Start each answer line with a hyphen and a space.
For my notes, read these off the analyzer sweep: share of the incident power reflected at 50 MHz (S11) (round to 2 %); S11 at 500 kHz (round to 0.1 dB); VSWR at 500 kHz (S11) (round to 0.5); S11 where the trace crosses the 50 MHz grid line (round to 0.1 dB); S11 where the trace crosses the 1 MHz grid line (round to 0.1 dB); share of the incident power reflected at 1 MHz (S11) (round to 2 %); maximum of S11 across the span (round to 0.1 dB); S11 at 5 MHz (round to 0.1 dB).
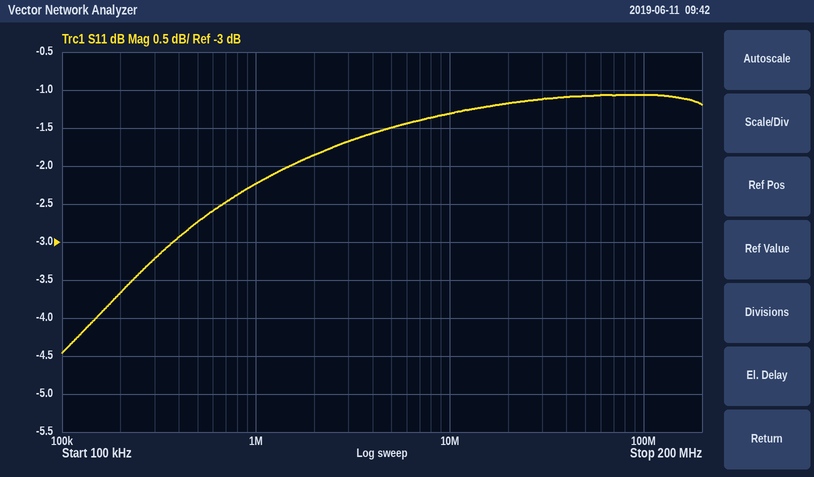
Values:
- 78 %
- -2.7 dB
- 6.5
- -1.1 dB
- -2.2 dB
- 60 %
- -1.1 dB
- -1.5 dB
